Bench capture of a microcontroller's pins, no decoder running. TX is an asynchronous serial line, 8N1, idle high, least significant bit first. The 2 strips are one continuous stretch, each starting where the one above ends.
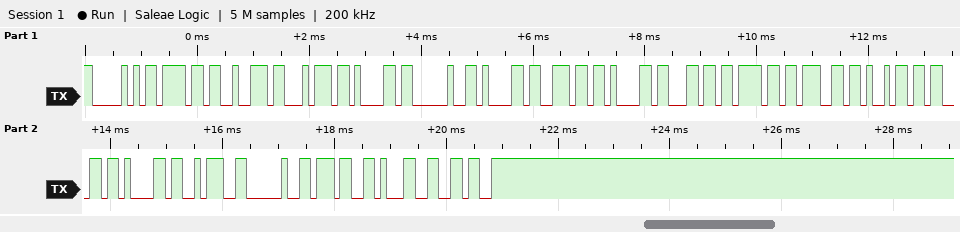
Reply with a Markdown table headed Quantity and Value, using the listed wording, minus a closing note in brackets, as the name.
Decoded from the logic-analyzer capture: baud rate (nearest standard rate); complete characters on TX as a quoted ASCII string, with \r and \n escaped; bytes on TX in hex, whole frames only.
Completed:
| Quantity | Value |
|---|---|
| baud rate | 9600 baud |
| complete characters on TX as a quoted ASCII string, with \r and \n escaped | "Porta analogica: 716" |
| bytes on TX in hex, whole frames only | 50 6F 72 74 61 20 61 6E 61 6C 6F 67 69 63 61 3A 20 37 31 36 |
